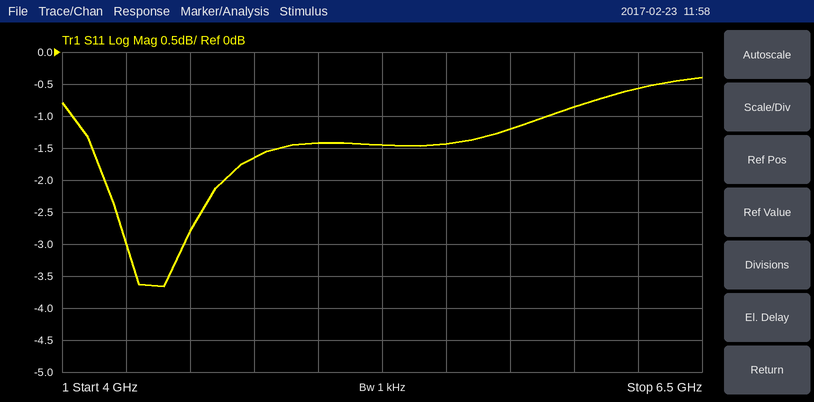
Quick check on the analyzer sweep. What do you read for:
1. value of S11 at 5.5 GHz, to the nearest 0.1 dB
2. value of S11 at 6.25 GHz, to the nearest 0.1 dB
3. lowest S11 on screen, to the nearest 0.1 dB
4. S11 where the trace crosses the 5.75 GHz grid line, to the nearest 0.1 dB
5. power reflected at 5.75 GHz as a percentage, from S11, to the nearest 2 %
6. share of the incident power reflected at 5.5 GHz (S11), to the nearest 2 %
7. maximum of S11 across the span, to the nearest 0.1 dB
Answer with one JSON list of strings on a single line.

["-1.4 dB", "-0.6 dB", "-3.7 dB", "-1.2 dB", "76 %", "72 %", "-0.4 dB"]
